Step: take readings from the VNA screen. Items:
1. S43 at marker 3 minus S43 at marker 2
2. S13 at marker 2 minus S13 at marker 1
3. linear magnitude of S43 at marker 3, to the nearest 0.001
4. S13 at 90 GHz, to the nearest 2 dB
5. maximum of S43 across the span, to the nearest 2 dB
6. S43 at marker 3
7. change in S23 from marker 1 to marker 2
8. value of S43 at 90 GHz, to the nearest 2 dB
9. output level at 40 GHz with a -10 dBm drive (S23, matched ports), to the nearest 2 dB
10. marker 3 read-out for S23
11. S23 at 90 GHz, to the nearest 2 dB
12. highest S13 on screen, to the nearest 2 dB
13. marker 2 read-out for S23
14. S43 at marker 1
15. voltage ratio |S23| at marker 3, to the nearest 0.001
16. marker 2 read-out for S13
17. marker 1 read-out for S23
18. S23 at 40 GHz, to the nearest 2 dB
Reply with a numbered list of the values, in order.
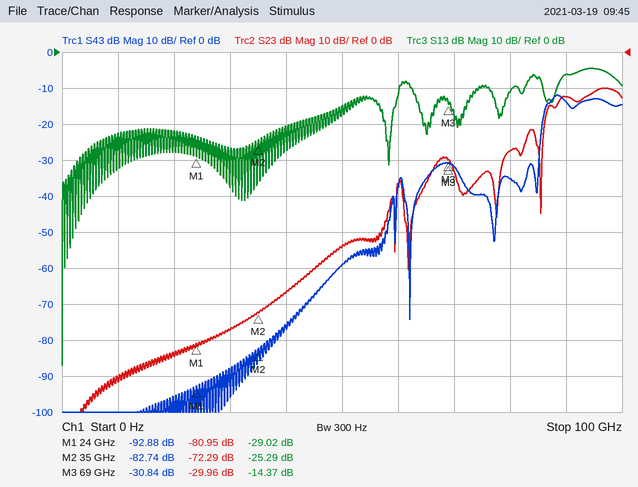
1. 51.90 dB
2. 3.73 dB
3. 0.029
4. -6 dB
5. -12 dB
6. -30.84 dB
7. 8.66 dB
8. -14 dB
9. -76 dBm
10. -29.96 dB
11. -12 dB
12. -4 dB
13. -72.29 dB
14. -92.88 dB
15. 0.032
16. -25.29 dB
17. -80.95 dB
18. -66 dB
